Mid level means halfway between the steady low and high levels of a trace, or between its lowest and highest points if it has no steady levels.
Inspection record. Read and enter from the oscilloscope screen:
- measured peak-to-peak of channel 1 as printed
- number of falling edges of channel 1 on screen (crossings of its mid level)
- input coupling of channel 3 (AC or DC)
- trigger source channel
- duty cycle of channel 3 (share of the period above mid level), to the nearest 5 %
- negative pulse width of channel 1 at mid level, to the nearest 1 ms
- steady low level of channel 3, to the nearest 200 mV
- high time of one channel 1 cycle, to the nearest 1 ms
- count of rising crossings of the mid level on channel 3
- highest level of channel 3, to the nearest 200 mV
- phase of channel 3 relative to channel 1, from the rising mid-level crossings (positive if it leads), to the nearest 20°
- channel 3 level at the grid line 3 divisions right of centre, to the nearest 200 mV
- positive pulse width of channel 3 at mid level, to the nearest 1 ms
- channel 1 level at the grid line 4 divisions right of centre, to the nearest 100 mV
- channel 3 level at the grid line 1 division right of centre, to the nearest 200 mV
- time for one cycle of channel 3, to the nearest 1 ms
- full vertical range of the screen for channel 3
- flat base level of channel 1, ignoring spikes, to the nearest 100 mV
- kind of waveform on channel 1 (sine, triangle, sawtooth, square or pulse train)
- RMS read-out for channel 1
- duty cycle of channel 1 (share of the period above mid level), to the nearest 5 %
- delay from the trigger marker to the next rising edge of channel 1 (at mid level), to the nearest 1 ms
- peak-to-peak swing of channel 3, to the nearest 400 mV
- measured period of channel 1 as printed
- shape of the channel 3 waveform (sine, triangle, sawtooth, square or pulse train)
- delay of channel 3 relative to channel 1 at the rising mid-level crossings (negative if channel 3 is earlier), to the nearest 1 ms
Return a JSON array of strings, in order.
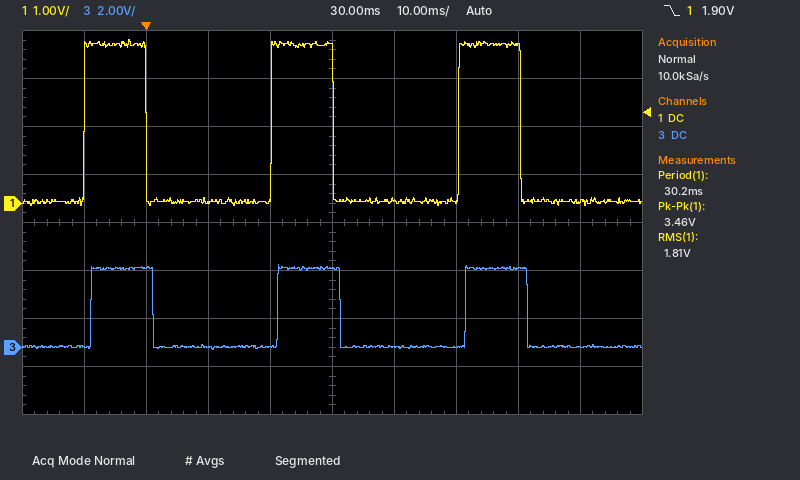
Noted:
["3.46 V", "3", "DC", "channel 1", "35 %", "20 ms", "0.0 V", "10 ms", "3", "3.4 V", "-20°", "3.2 V", "10 ms", "0.0 V", "0.0 V", "30 ms", "16 V", "0.0 V", "pulse train", "1.81 V", "35 %", "20 ms", "3.6 V", "30.2 ms", "pulse train", "+1 ms"]
